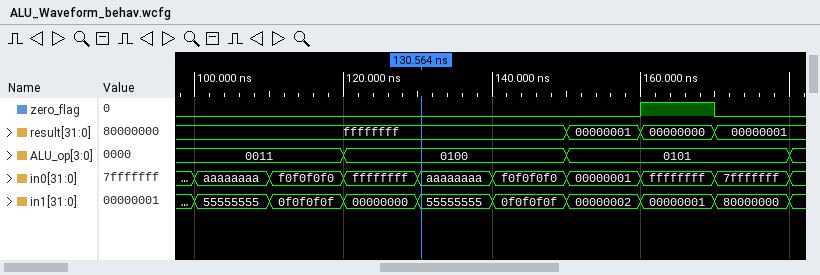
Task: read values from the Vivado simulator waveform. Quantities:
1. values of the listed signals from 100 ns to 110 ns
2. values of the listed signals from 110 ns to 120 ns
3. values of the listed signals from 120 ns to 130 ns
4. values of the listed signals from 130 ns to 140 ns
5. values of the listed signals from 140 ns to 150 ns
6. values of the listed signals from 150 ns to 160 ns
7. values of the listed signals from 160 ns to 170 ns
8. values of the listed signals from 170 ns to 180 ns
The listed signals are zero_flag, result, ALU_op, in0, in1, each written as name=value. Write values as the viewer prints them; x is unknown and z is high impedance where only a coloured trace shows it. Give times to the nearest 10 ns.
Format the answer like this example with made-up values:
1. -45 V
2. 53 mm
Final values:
1. zero_flag=0, result=ffffffff, ALU_op=0011, in0=aaaaaaaa, in1=55555555
2. zero_flag=0, result=ffffffff, ALU_op=0011, in0=f0f0f0f0, in1=0f0f0f0f
3. zero_flag=0, result=ffffffff, ALU_op=0100, in0=ffffffff, in1=00000000
4. zero_flag=0, result=ffffffff, ALU_op=0100, in0=aaaaaaaa, in1=55555555
5. zero_flag=0, result=ffffffff, ALU_op=0100, in0=f0f0f0f0, in1=0f0f0f0f
6. zero_flag=0, result=00000001, ALU_op=0101, in0=00000001, in1=00000002
7. zero_flag=1, result=00000000, ALU_op=0101, in0=ffffffff, in1=00000001
8. zero_flag=0, result=00000001, ALU_op=0101, in0=7fffffff, in1=80000000
